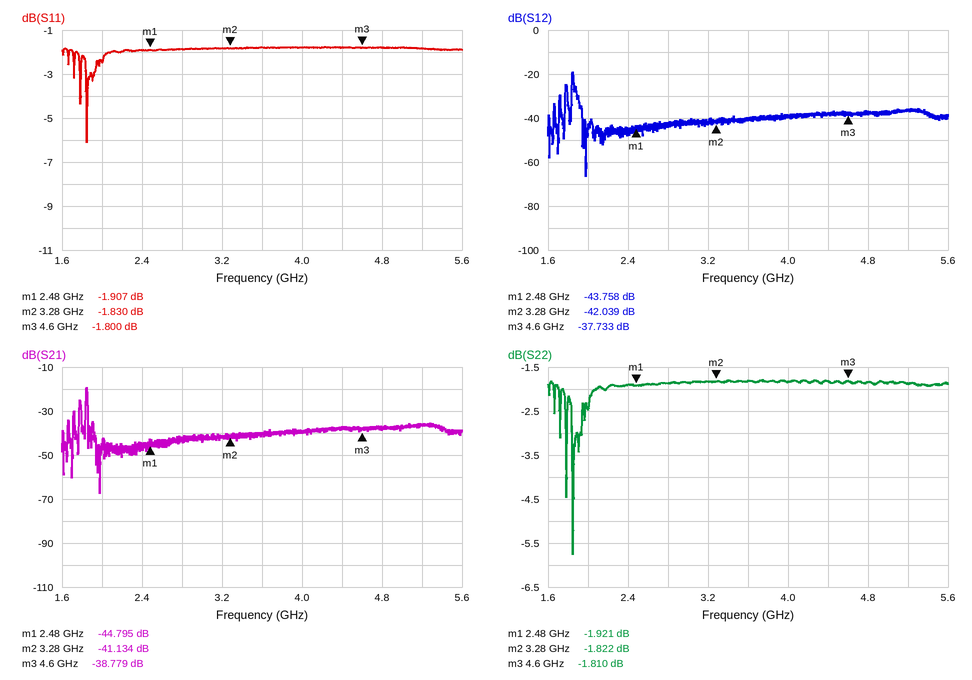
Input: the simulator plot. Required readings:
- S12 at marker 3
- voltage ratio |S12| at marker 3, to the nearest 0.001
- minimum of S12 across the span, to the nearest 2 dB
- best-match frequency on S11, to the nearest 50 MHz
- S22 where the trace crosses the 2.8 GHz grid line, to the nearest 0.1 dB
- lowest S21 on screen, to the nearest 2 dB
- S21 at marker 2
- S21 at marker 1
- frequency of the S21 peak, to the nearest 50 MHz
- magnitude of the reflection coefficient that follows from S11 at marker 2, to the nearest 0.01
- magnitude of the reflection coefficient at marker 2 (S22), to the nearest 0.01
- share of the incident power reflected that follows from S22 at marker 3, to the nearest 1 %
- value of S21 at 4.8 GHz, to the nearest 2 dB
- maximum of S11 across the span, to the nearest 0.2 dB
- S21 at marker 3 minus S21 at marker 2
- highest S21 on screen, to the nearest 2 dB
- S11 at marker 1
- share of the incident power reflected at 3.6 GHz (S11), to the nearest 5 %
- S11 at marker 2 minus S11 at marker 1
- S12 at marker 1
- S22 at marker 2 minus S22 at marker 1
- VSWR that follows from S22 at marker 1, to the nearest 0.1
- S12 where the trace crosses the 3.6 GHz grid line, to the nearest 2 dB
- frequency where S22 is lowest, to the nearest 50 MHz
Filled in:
-37.733 dB
0.013
-66 dB
1.85 GHz
-1.9 dB
-68 dB
-41.134 dB
-44.795 dB
1.85 GHz
0.81
0.81
66 %
-38 dB
-1.8 dB
2.355 dB
-20 dB
-1.907 dB
65 %
0.077 dB
-43.758 dB
0.099 dB
9.1
-40 dB
1.85 GHz
